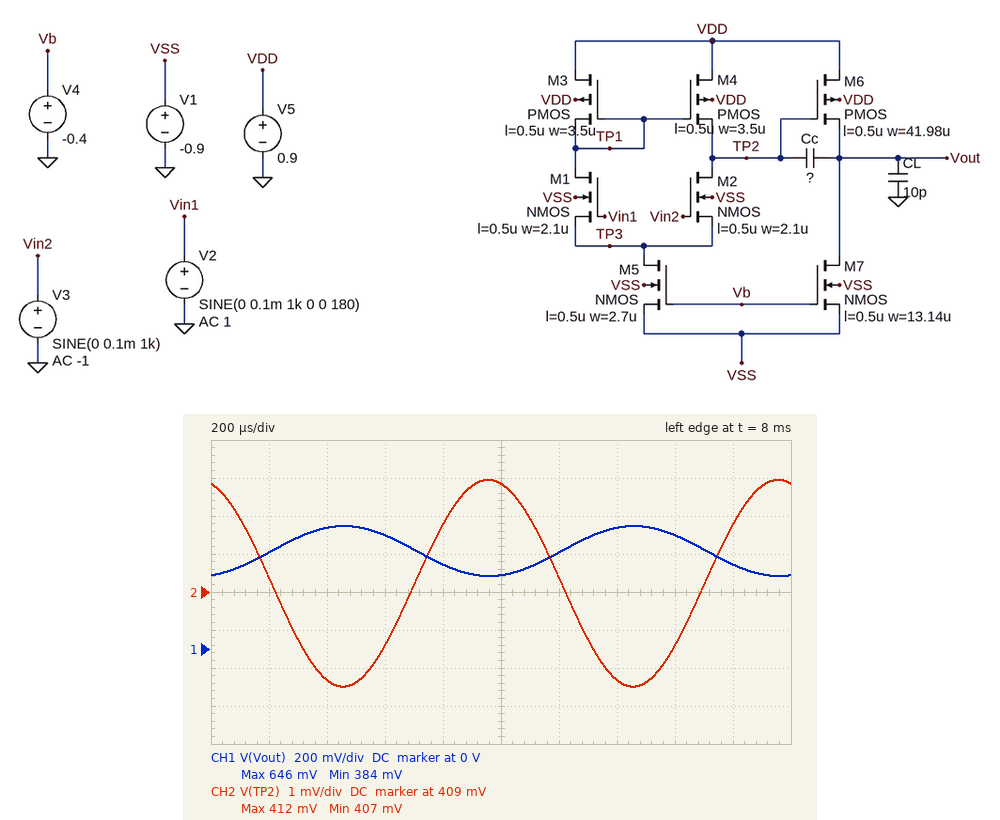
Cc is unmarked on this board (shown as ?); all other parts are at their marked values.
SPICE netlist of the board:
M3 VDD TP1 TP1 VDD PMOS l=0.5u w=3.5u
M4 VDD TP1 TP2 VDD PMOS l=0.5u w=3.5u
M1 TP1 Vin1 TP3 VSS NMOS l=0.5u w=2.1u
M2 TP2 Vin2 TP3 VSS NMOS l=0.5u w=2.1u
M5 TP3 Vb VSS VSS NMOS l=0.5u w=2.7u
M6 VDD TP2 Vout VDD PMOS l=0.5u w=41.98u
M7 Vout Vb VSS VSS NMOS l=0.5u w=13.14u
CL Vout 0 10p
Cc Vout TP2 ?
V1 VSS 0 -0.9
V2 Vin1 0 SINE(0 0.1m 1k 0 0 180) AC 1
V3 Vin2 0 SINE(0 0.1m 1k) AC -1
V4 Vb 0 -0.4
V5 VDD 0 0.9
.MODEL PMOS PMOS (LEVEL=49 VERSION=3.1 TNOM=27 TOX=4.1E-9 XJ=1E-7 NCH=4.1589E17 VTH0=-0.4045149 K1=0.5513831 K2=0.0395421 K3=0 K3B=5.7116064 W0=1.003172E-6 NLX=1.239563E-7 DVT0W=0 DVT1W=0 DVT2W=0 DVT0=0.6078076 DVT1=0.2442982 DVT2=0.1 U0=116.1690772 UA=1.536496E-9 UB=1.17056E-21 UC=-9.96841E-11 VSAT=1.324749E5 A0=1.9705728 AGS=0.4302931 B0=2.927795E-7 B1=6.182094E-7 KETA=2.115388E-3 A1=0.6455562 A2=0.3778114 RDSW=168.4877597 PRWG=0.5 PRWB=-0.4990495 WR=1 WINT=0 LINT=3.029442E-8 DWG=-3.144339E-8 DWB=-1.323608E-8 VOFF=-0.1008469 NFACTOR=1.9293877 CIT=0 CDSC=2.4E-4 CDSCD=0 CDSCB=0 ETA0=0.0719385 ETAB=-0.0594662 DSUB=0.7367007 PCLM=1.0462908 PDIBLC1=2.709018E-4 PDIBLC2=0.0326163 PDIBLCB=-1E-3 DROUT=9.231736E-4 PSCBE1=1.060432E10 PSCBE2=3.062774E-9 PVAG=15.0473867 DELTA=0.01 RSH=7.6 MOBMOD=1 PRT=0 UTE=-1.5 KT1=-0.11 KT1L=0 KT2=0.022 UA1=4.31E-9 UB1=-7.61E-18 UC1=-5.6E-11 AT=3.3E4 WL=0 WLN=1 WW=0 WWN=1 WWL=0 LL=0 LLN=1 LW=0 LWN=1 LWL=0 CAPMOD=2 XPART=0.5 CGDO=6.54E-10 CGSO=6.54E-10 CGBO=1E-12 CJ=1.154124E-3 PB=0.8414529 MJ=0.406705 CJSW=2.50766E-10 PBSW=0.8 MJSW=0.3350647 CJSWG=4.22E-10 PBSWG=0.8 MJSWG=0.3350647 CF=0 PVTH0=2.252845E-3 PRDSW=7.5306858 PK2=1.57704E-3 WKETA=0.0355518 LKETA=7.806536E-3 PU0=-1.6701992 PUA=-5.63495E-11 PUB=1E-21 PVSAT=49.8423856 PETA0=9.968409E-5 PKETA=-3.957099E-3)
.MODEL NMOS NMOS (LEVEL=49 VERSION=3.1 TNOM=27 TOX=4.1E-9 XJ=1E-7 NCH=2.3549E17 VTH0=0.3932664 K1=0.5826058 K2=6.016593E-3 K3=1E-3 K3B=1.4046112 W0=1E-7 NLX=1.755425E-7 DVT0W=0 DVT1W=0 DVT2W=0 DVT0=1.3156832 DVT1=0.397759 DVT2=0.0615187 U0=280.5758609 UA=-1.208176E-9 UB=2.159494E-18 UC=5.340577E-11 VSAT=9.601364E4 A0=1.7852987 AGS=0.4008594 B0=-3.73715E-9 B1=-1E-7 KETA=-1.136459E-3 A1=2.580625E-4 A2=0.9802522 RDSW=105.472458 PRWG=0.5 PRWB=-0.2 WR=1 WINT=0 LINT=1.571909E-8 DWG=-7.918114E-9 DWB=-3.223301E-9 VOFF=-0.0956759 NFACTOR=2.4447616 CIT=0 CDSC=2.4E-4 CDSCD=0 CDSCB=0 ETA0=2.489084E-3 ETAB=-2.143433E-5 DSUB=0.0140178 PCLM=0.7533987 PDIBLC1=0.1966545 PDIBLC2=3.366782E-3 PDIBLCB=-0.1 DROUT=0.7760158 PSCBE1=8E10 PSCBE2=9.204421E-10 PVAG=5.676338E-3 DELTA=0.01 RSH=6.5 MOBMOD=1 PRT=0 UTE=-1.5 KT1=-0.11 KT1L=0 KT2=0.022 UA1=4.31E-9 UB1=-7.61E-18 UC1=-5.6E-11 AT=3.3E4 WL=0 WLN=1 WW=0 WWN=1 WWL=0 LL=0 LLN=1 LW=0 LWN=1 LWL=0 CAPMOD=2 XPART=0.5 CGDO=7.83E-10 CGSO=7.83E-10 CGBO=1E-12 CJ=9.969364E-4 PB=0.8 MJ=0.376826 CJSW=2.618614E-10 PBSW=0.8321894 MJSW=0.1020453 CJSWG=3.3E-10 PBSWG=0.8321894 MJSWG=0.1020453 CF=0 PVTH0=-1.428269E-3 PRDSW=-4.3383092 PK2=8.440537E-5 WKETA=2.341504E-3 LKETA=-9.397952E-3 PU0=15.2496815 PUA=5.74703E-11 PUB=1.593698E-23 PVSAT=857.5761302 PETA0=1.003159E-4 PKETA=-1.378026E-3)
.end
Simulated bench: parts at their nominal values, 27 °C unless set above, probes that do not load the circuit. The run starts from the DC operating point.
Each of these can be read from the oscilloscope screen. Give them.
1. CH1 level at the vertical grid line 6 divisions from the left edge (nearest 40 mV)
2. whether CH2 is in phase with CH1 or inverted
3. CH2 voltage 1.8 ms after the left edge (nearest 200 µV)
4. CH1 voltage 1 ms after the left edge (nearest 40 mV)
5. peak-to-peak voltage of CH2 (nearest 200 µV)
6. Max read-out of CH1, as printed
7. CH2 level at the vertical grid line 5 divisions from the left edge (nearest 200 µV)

520 mV
inverted
410.8 mV
400 mV
5.4 mV
646 mV
411.8 mV
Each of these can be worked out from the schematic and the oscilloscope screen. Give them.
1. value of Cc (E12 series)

4.7 pF
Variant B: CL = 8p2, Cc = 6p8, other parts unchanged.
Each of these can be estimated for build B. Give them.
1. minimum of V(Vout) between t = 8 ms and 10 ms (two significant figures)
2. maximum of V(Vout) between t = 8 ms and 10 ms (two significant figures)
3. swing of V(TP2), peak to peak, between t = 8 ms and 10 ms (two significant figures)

420 mV
610 mV
3.8 mV
